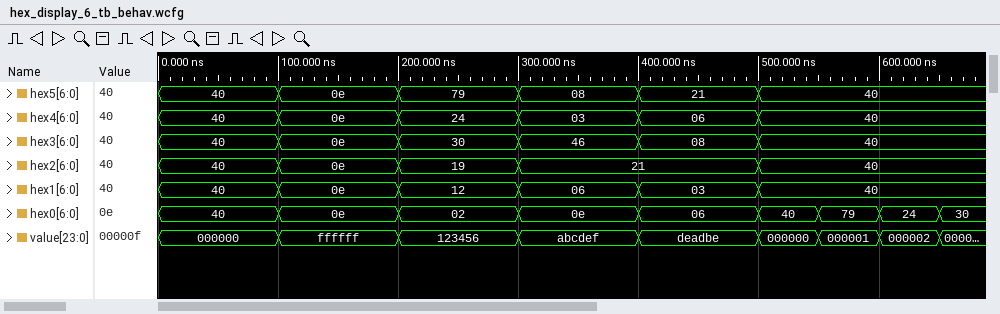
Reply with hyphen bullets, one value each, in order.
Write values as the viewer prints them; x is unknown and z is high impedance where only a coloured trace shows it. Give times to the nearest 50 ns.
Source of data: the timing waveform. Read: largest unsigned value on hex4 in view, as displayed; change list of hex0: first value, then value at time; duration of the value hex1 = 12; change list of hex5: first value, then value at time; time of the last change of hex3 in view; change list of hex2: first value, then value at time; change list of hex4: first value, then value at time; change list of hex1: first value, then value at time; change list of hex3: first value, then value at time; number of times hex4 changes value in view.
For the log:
- 40
- 40, 0e at 100 ns, 02 at 200 ns, 0e at 300 ns, 06 at 400 ns, 40 at 500 ns, 79 at 550 ns, 24 at 600 ns, 30 at 650 ns
- 100 ns
- 40, 0e at 100 ns, 79 at 200 ns, 08 at 300 ns, 21 at 400 ns, 40 at 500 ns
- 500 ns
- 40, 0e at 100 ns, 19 at 200 ns, 21 at 300 ns, 40 at 500 ns
- 40, 0e at 100 ns, 24 at 200 ns, 03 at 300 ns, 06 at 400 ns, 40 at 500 ns
- 40, 0e at 100 ns, 12 at 200 ns, 06 at 300 ns, 03 at 400 ns, 40 at 500 ns
- 40, 0e at 100 ns, 30 at 200 ns, 46 at 300 ns, 08 at 400 ns, 40 at 500 ns
- 5
